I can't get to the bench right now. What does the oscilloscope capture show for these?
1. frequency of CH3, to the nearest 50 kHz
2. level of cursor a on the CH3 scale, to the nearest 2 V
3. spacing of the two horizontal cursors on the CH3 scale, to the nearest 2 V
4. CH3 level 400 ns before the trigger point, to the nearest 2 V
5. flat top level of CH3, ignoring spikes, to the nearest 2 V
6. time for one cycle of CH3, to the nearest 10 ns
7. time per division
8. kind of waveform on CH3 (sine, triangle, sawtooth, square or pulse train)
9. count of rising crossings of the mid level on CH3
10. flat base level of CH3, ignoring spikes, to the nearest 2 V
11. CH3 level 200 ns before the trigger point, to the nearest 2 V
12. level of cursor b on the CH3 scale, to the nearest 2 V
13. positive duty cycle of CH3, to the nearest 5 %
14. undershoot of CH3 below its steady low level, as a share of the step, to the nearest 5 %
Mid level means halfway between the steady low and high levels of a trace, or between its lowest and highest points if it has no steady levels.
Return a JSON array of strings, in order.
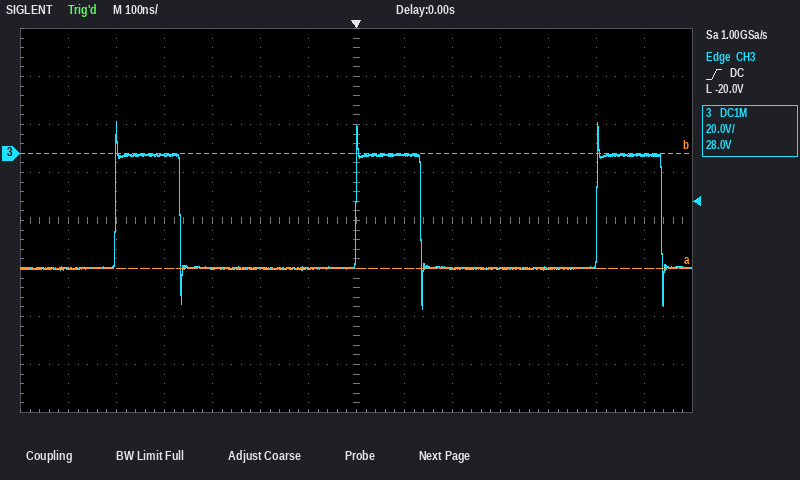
["2.00 MHz", "-48 V", "48 V", "0 V", "0 V", "500 ns", "100 ns", "pulse train", "3", "-48 V", "-48 V", "0 V", "25 %", "35 %"]
